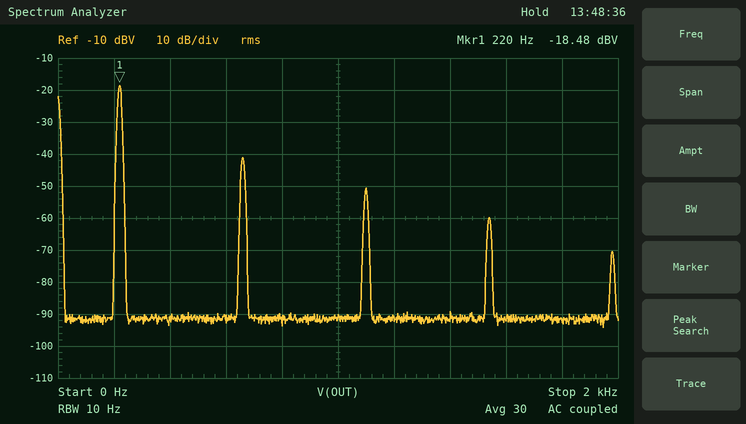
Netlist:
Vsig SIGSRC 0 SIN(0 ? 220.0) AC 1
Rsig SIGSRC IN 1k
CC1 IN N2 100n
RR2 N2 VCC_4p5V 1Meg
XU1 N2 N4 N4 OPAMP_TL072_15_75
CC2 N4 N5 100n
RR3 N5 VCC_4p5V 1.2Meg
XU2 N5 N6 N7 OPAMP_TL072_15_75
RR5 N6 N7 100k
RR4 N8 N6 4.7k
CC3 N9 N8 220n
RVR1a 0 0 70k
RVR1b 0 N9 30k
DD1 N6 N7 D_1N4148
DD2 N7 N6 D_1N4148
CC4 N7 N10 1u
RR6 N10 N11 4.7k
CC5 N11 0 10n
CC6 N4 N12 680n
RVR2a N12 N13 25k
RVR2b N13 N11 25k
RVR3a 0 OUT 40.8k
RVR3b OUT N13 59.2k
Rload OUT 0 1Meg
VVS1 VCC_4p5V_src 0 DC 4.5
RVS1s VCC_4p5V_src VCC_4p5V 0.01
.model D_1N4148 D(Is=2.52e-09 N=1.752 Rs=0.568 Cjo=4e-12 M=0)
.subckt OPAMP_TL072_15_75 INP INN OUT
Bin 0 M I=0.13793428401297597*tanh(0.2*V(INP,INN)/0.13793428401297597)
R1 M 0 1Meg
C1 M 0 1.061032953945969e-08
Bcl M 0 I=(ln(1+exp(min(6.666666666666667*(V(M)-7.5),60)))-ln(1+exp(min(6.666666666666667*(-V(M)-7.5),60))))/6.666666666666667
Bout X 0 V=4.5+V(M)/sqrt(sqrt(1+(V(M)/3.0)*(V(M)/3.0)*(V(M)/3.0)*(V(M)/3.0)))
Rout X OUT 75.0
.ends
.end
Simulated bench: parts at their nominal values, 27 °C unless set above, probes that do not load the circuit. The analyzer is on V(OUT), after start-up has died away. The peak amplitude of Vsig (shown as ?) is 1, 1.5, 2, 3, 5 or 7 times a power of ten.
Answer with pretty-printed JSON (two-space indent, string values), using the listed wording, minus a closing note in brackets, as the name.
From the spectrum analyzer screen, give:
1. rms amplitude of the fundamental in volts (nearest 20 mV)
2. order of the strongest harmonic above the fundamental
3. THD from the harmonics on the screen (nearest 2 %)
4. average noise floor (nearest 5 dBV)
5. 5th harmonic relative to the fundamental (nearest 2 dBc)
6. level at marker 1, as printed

{
  "rms amplitude of the fundamental in volts": "120 mV",
  "order of the strongest harmonic above the fundamental": "3",
  "THD from the harmonics on the screen": "8 %",
  "average noise floor": "-90 dBV",
  "5th harmonic relative to the fundamental": "-32 dBc",
  "level at marker 1, as printed": "-18.48 dBV"
}
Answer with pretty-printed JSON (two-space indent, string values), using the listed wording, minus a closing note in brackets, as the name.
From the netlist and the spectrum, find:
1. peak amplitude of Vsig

{
  "peak amplitude of Vsig": "300 mV"
}
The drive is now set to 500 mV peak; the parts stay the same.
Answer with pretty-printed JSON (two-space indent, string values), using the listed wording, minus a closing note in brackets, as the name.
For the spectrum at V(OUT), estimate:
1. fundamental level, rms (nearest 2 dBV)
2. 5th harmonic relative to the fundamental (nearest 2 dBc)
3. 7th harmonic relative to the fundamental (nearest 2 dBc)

{
  "fundamental level, rms": "-16 dBV",
  "5th harmonic relative to the fundamental": "-30 dBc",
  "7th harmonic relative to the fundamental": "-36 dBc"
}
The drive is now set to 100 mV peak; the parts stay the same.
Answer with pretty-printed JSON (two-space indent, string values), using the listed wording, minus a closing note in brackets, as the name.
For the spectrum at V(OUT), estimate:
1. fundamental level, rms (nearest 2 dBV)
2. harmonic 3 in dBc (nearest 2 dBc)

{
  "fundamental level, rms": "-26 dBV",
  "harmonic 3 in dBc": "-32 dBc"
}
